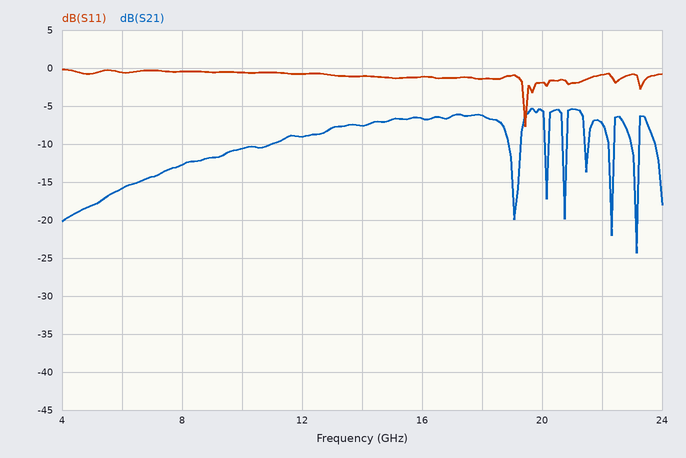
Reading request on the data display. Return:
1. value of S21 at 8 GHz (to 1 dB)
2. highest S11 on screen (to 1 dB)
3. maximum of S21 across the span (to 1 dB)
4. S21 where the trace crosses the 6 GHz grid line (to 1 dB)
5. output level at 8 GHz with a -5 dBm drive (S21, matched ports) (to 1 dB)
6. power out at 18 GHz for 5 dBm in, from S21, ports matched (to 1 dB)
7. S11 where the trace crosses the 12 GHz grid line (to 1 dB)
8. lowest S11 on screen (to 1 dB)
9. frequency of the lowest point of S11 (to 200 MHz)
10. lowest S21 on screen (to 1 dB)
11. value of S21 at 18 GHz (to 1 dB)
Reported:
-13 dB
0 dB
-5 dB
-16 dB
-18 dBm
-1 dBm
-1 dB
-8 dB
19.4 GHz
-24 dB
-6 dB
